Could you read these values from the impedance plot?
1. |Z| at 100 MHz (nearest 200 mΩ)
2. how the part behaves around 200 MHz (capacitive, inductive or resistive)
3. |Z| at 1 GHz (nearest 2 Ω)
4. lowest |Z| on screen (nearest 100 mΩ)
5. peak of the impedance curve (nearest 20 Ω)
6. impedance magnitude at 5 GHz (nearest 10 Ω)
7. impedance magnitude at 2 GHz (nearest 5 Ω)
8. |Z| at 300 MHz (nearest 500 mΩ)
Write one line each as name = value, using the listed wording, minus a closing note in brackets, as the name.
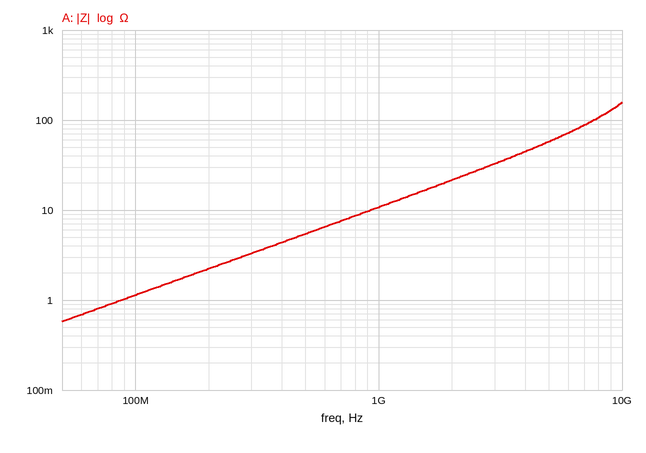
|Z| at 100 MHz = 1.2 Ω
how the part behaves around 200 MHz = inductive
|Z| at 1 GHz = 10 Ω
lowest |Z| on screen = 600 mΩ
peak of the impedance curve = 160 Ω
impedance magnitude at 5 GHz = 60 Ω
impedance magnitude at 2 GHz = 20 Ω
|Z| at 300 MHz = 3.5 Ω
